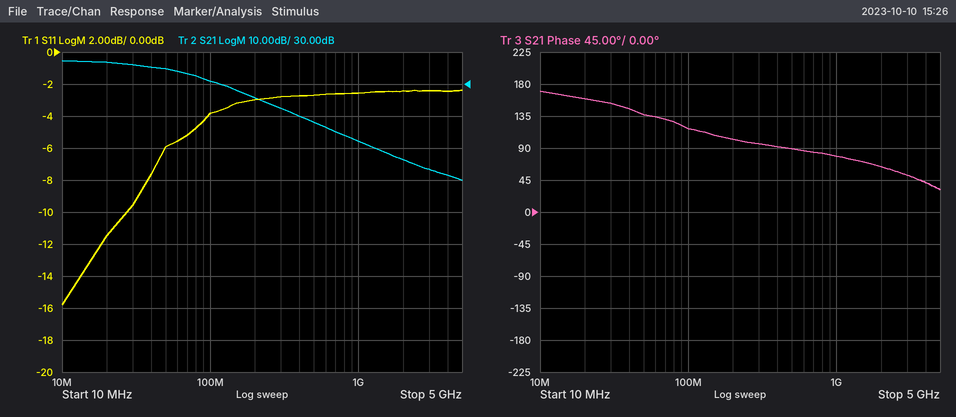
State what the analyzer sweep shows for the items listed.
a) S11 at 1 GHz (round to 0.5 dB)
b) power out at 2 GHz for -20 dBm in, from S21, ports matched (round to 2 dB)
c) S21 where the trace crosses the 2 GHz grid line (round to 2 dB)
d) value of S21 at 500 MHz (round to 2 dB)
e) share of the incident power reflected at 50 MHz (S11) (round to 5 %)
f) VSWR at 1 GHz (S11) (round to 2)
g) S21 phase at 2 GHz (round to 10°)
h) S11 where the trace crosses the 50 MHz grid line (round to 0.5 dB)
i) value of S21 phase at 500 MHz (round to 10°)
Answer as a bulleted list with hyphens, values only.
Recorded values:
- -2.5 dB
- -14 dBm
- 6 dB
- 18 dB
- 25 %
- 6
- 60°
- -6.0 dB
- 90°
